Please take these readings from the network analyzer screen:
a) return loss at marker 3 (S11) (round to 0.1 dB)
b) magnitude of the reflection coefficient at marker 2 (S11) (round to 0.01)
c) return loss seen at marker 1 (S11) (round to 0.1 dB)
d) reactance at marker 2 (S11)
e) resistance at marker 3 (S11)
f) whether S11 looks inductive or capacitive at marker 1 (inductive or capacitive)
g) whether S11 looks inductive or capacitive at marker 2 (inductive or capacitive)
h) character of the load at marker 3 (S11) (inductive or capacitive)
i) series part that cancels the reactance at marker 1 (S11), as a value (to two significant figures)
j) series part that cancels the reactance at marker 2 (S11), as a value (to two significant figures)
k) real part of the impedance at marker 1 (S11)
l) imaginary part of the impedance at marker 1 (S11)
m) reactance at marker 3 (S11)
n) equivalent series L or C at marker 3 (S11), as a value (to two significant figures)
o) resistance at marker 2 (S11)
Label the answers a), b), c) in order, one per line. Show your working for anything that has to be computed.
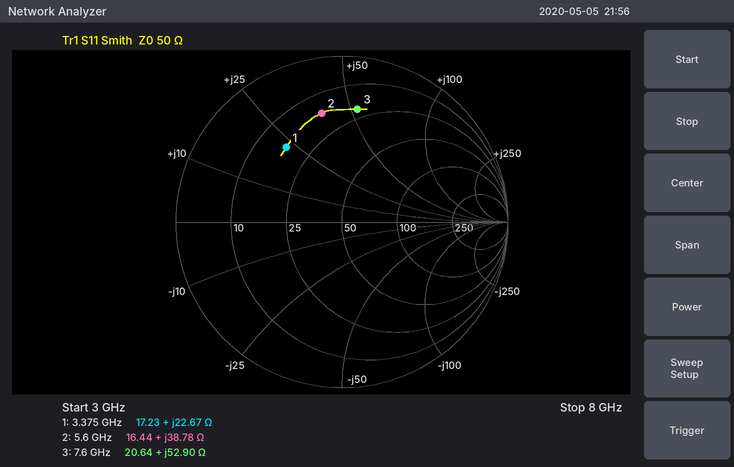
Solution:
a) 3.3 dB
b) 0.67
c) 5.0 dB
d) +38.78 Ω
e) 20.64 Ω
f) inductive
g) inductive
h) inductive
i) C = 1/(2π × 3.375 GHz × 22.67 Ω) ≈ 2.1 pF
j) C = 1/(2π × 5.6 GHz × 38.78 Ω) ≈ 733 fF, so 730 fF to two significant figures
k) 17.23 Ω
l) +22.67 Ω
m) +52.90 Ω
n) L = 52.9 Ω/(2π × 7.6 GHz) ≈ 1.1 nH
o) 16.44 Ω
